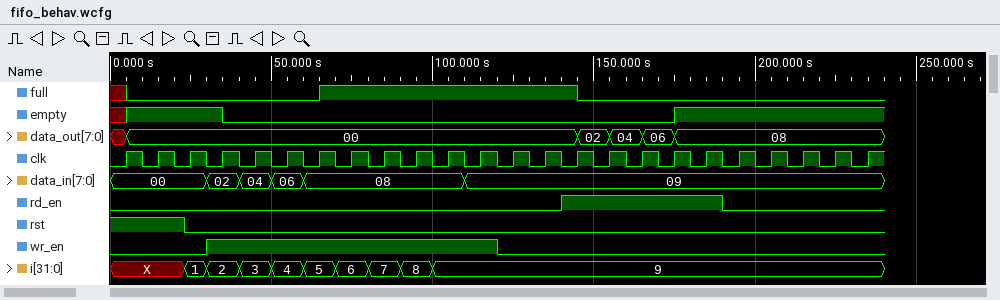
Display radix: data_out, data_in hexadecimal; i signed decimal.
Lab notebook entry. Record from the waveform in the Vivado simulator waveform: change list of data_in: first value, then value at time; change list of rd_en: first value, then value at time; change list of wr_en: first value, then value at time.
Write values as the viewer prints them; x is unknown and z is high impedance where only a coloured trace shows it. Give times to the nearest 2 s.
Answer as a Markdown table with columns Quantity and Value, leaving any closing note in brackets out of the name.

| Quantity | Value |
|---|---|
| change list of data_in: first value, then value at time | 00, 02 at 30 s, 04 at 40 s, 06 at 50 s, 08 at 60 s, 09 at 110 s |
| change list of rd_en: first value, then value at time | 0, 1 at 140 s, 0 at 190 s |
| change list of wr_en: first value, then value at time | 0, 1 at 30 s, 0 at 120 s |
